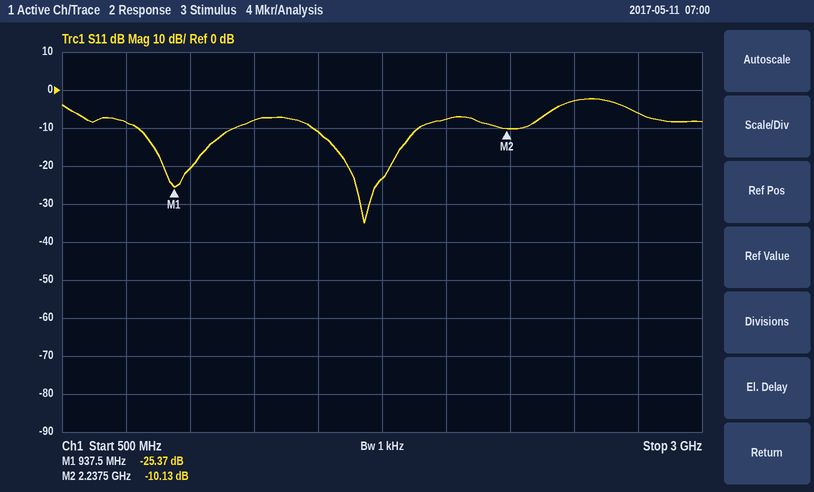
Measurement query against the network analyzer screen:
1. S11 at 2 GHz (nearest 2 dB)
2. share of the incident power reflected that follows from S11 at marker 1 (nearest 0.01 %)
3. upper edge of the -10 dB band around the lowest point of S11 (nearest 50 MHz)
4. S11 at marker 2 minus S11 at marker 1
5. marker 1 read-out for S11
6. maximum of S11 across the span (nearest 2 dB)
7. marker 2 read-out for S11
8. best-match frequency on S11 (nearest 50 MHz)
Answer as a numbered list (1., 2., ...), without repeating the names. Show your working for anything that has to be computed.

1. -8 dB
2. 10^(-25.37/10) ≈ 0.29 %
3. 1.90 GHz
4. -10.13 − (-25.37) = 15.24 dB
5. -25.37 dB
6. -2 dB
7. -10.13 dB
8. 1.70 GHz
